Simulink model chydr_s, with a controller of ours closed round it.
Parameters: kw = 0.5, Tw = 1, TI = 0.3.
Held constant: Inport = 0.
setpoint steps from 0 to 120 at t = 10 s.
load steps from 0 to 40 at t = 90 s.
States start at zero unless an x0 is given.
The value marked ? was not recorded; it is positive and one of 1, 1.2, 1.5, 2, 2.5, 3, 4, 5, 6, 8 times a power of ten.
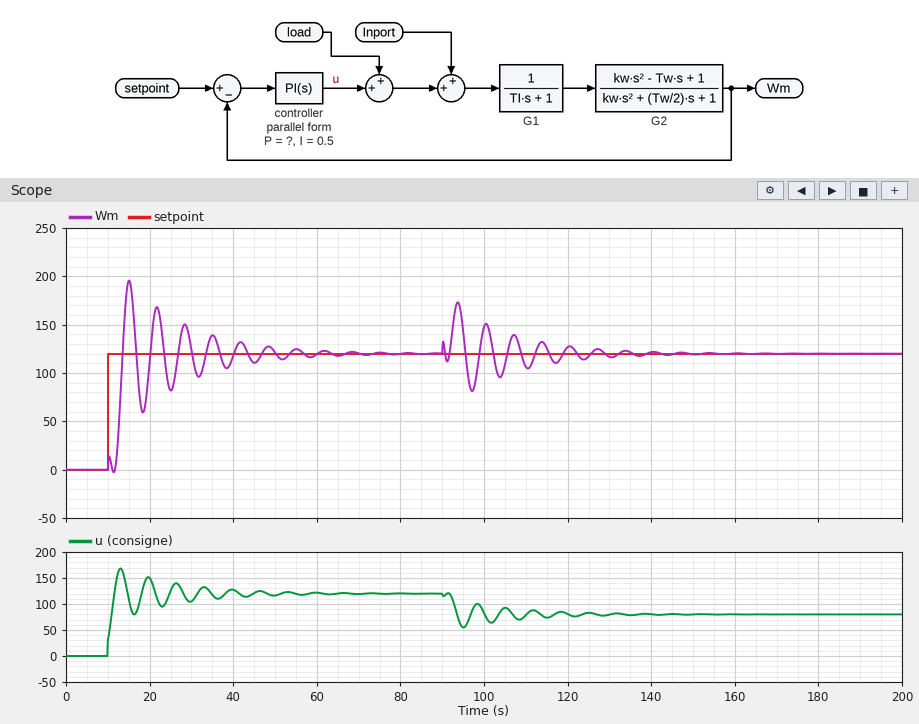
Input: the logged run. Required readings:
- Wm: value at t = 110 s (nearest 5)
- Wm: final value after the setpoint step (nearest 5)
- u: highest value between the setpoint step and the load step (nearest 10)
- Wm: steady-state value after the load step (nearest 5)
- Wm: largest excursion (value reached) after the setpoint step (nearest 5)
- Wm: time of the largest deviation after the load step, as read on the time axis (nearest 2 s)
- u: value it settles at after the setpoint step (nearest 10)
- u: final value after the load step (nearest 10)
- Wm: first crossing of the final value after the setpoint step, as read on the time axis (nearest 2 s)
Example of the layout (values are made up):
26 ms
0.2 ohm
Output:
105
120
170
120
195
94 s
120
80
14 s
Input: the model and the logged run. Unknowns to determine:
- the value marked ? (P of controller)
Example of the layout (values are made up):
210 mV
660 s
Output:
0.25
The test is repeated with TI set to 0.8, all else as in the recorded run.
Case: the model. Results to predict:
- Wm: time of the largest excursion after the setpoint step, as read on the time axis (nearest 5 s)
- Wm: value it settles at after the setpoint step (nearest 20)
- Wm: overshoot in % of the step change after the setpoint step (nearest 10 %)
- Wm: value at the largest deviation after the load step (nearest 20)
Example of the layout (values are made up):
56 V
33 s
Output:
15 s
120
60 %
160
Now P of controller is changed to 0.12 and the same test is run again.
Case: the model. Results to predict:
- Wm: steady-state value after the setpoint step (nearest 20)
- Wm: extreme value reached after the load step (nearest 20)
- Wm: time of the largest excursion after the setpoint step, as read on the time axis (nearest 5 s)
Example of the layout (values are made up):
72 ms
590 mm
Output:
120
180
15 s
